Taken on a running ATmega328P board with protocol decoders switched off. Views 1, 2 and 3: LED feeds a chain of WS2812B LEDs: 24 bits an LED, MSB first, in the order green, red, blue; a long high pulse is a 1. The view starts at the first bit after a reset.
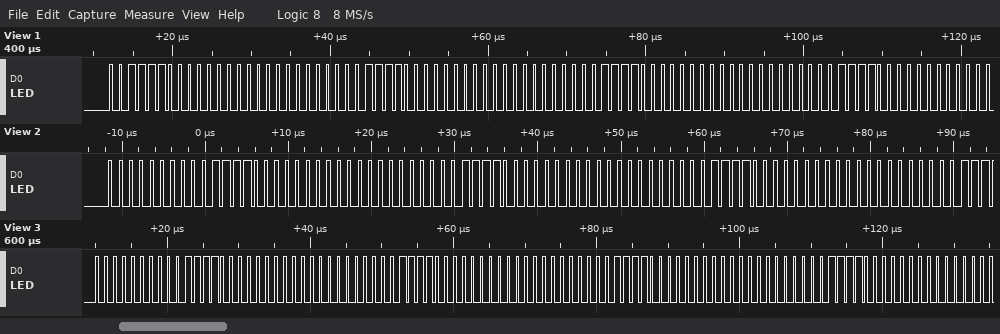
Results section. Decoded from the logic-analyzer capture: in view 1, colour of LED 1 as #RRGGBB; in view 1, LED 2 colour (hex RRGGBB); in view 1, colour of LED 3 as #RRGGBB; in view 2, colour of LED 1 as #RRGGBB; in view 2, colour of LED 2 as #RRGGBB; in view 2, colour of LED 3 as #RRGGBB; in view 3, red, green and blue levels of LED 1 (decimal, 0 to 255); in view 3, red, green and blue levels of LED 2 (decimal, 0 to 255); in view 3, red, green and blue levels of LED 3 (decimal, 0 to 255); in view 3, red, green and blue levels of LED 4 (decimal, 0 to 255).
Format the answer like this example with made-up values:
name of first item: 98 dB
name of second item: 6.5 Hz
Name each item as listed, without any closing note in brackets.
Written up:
in view 1, colour of LED 1 as #RRGGBB: #003C00
in view 1, LED 2 colour: #003C00
in view 1, colour of LED 3 as #RRGGBB: #003C00
in view 2, colour of LED 1 as #RRGGBB: #3C0000
in view 2, colour of LED 2 as #RRGGBB: #3C0000
in view 2, colour of LED 3 as #RRGGBB: #3C0000
in view 3, red, green and blue levels of LED 1: 60, 0, 0
in view 3, red, green and blue levels of LED 2: 60, 0, 0
in view 3, red, green and blue levels of LED 3: 60, 0, 0
in view 3, red, green and blue levels of LED 4: 60, 0, 0
